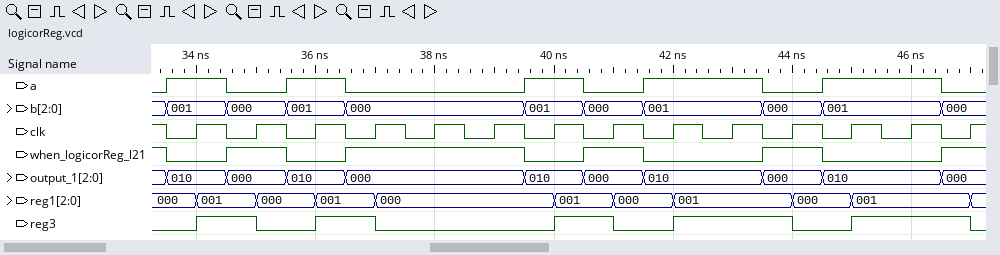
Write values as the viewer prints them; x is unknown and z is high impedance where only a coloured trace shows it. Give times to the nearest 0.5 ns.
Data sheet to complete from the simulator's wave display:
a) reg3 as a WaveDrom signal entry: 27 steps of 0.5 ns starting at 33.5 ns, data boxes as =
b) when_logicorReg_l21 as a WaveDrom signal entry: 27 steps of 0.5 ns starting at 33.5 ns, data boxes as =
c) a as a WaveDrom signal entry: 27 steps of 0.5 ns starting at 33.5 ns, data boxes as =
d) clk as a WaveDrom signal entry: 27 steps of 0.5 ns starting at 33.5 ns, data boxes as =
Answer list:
{name: 'reg3', wave: '01.0.1.0.....1.0.1...0.1...'}
{name: 'when_logicorReg_l21', wave: '0.1.0.1.....0.1.0...1.0...1'}
{name: 'a', wave: '1.0.1.0.....1.0.1...0.1...0'}
{name: 'clk', wave: '010101010101010101010101010'}
